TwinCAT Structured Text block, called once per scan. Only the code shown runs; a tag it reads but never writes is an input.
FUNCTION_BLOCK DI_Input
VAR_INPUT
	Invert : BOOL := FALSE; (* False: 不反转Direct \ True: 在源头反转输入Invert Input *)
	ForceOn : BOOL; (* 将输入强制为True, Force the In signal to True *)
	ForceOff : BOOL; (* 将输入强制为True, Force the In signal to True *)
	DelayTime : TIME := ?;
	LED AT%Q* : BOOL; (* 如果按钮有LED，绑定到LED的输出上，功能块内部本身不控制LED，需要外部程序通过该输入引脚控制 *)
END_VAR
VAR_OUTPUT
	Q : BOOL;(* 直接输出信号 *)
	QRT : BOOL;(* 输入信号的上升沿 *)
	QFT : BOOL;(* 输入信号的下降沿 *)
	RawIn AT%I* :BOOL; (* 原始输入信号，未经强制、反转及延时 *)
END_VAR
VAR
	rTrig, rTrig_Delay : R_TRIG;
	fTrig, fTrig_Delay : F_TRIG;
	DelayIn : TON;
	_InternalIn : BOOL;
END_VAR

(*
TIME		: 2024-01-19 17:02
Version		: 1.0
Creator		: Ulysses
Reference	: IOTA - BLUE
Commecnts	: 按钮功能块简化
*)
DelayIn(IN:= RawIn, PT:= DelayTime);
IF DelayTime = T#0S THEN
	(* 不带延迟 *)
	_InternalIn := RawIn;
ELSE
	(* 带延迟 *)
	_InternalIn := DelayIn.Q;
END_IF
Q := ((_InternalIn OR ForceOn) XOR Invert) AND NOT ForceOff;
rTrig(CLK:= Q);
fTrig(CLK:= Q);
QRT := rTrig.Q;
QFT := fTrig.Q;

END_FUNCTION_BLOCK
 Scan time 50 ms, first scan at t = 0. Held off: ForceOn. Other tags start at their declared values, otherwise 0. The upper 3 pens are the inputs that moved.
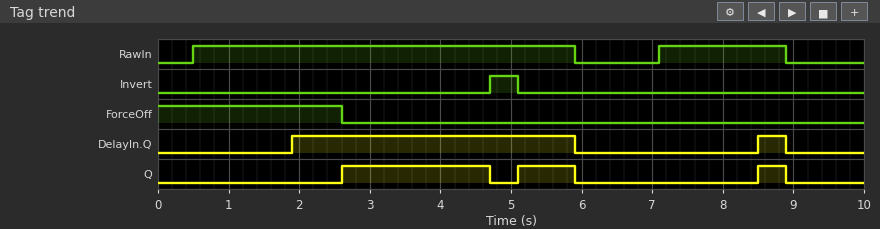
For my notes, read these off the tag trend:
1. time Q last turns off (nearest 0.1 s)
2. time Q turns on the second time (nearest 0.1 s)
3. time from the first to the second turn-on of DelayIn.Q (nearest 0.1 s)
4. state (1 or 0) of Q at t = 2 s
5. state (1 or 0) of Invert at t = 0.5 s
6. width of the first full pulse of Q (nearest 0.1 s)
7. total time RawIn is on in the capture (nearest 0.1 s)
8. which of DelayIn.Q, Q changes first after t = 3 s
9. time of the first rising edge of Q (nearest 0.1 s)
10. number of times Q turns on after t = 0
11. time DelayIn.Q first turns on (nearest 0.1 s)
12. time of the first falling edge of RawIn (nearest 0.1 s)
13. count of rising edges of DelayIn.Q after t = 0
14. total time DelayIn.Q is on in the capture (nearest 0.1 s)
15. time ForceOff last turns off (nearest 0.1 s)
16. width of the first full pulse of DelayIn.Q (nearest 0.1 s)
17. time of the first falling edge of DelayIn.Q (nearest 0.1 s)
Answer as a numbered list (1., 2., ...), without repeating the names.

1. 8.9 s
2. 5.1 s
3. 6.6 s
4. 0
5. 0
6. 2.1 s
7. 7.2 s
8. Q
9. 2.6 s
10. 3
11. 1.9 s
12. 5.9 s
13. 2
14. 4.4 s
15. 2.6 s
16. 4.0 s
17. 5.9 s
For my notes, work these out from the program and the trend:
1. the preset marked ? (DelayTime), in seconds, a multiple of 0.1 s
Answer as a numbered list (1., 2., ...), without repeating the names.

1. 1.4 s
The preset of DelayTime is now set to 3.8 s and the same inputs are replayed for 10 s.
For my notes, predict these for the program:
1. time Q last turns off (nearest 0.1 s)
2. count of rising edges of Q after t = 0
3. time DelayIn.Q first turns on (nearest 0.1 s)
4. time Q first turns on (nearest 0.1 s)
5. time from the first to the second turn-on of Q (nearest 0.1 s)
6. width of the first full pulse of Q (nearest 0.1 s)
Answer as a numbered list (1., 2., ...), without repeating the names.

1. 5.9 s
2. 2
3. 4.3 s
4. 4.3 s
5. 0.8 s
6. 0.4 s
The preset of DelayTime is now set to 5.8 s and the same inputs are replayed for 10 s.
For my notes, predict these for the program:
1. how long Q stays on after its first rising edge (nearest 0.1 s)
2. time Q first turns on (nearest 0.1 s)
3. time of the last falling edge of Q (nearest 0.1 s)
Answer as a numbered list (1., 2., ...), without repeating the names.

1. 0.4 s
2. 4.7 s
3. 5.1 s
